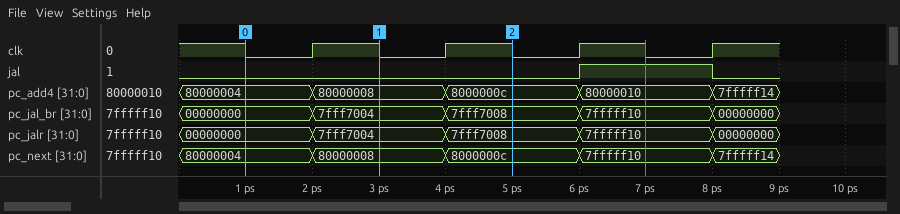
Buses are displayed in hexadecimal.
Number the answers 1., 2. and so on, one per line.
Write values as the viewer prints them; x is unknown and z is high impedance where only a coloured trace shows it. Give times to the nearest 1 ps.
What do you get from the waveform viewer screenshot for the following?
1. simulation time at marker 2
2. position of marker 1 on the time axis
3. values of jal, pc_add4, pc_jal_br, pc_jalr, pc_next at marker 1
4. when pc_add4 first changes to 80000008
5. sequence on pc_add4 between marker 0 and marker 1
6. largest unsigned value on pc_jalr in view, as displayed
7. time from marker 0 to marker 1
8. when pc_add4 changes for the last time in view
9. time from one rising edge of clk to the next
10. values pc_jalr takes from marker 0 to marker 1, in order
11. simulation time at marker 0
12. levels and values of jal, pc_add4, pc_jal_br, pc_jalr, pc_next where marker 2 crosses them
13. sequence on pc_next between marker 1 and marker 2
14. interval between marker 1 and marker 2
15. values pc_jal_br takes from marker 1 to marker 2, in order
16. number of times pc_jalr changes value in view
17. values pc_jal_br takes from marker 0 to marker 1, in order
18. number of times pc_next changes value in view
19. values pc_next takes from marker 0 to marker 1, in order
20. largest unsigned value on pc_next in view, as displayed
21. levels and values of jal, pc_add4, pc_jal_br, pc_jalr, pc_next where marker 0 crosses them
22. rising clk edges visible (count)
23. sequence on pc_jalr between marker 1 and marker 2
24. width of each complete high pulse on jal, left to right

1. 5 ps
2. 3 ps
3. jal=0, pc_add4=80000008, pc_jal_br=7fff7004, pc_jalr=7fff7004, pc_next=80000008
4. 2 ps
5. 80000004, 80000008
6. 7fffff10
7. 2 ps
8. 8 ps
9. 2 ps
10. 00000000, 7fff7004
11. 1 ps
12. jal=0, pc_add4=8000000c, pc_jal_br=7fff7008, pc_jalr=7fff7008, pc_next=8000000c
13. 80000008, 8000000c
14. 2 ps
15. 7fff7004, 7fff7008
16. 4
17. 00000000, 7fff7004
18. 4
19. 80000004, 80000008
20. 8000000c
21. jal=0, pc_add4=80000004, pc_jal_br=00000000, pc_jalr=00000000, pc_next=80000004
22. 4
23. 7fff7004, 7fff7008
24. 2 ps
